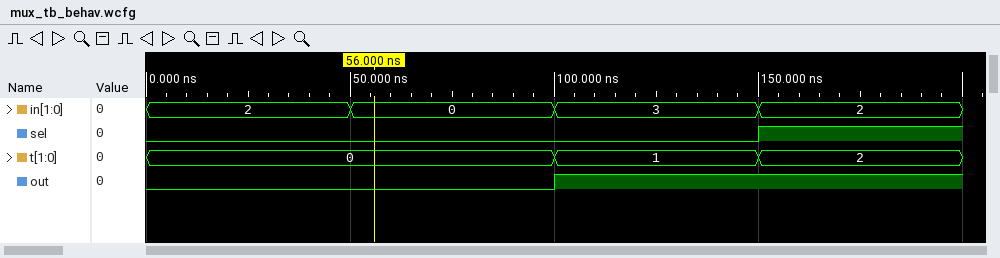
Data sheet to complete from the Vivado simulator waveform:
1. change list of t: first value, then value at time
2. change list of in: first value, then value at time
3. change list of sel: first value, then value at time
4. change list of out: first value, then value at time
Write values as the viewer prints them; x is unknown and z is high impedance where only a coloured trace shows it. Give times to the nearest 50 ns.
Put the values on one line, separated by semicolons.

0, 1 at 100 ns, 2 at 150 ns; 2, 0 at 50 ns, 3 at 100 ns, 2 at 150 ns; 0, 1 at 150 ns; 0, 1 at 100 ns
